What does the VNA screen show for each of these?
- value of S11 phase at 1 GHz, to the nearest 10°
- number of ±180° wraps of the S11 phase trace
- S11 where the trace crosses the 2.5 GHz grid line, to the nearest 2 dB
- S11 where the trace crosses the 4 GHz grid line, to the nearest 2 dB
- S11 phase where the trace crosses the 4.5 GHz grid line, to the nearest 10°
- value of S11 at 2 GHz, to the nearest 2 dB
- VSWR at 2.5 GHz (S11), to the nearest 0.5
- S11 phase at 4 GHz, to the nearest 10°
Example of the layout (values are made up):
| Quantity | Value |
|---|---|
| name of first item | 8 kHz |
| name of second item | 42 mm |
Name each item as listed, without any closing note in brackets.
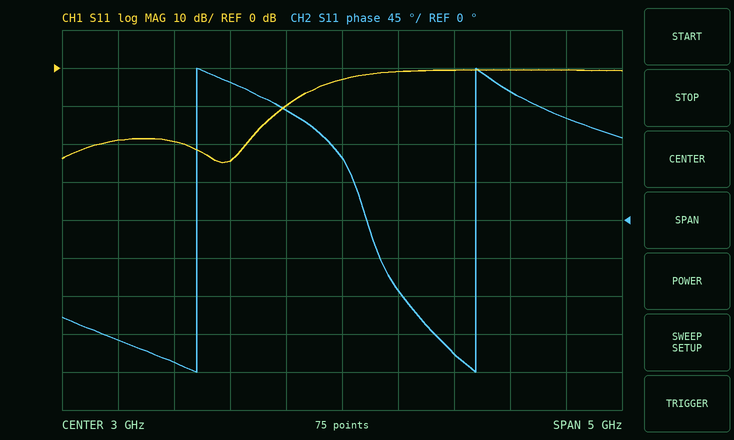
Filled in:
| Quantity | Value |
|---|---|
| value of S11 phase at 1 GHz, to the nearest 10° | -140° |
| number of ±180° wraps of the S11 phase trace | 2 |
| S11 where the trace crosses the 2.5 GHz grid line, to the nearest 2 dB | -10 dB |
| S11 where the trace crosses the 4 GHz grid line, to the nearest 2 dB | 0 dB |
| S11 phase where the trace crosses the 4.5 GHz grid line, to the nearest 10° | 150° |
| value of S11 at 2 GHz, to the nearest 2 dB | -24 dB |
| VSWR at 2.5 GHz (S11), to the nearest 0.5 | 2.0 |
| S11 phase at 4 GHz, to the nearest 10° | -160° |
